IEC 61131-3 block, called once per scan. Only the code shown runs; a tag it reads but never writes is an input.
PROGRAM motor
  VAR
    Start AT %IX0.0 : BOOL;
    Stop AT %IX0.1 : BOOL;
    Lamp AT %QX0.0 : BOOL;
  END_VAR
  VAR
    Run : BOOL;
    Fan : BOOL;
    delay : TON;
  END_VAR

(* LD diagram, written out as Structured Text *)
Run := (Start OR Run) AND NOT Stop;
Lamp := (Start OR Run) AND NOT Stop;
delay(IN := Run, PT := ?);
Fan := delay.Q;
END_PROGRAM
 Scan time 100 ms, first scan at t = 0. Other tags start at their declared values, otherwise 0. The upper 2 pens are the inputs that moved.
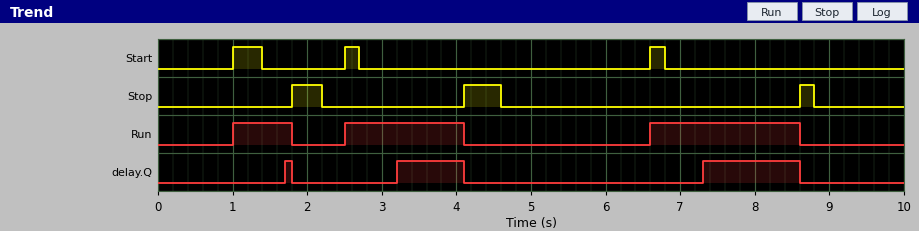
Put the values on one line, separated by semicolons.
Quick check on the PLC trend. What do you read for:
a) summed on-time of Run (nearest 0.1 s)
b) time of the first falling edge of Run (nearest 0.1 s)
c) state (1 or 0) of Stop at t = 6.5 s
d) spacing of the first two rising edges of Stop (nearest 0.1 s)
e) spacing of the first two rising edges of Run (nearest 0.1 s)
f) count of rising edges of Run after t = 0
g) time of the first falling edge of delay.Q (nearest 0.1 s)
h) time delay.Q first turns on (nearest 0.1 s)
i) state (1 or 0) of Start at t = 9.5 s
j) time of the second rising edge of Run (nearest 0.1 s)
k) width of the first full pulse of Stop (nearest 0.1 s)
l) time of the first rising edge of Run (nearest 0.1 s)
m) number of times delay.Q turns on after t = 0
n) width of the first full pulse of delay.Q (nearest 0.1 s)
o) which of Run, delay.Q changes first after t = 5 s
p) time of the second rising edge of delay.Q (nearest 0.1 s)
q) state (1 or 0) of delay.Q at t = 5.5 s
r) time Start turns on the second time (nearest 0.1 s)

4.4 s; 1.8 s; 0; 2.3 s; 1.5 s; 3; 1.8 s; 1.7 s; 0; 2.5 s; 0.4 s; 1.0 s; 3; 0.1 s; Run; 3.2 s; 0; 2.5 s
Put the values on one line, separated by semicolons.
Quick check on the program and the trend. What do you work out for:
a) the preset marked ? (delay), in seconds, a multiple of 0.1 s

0.7 s
